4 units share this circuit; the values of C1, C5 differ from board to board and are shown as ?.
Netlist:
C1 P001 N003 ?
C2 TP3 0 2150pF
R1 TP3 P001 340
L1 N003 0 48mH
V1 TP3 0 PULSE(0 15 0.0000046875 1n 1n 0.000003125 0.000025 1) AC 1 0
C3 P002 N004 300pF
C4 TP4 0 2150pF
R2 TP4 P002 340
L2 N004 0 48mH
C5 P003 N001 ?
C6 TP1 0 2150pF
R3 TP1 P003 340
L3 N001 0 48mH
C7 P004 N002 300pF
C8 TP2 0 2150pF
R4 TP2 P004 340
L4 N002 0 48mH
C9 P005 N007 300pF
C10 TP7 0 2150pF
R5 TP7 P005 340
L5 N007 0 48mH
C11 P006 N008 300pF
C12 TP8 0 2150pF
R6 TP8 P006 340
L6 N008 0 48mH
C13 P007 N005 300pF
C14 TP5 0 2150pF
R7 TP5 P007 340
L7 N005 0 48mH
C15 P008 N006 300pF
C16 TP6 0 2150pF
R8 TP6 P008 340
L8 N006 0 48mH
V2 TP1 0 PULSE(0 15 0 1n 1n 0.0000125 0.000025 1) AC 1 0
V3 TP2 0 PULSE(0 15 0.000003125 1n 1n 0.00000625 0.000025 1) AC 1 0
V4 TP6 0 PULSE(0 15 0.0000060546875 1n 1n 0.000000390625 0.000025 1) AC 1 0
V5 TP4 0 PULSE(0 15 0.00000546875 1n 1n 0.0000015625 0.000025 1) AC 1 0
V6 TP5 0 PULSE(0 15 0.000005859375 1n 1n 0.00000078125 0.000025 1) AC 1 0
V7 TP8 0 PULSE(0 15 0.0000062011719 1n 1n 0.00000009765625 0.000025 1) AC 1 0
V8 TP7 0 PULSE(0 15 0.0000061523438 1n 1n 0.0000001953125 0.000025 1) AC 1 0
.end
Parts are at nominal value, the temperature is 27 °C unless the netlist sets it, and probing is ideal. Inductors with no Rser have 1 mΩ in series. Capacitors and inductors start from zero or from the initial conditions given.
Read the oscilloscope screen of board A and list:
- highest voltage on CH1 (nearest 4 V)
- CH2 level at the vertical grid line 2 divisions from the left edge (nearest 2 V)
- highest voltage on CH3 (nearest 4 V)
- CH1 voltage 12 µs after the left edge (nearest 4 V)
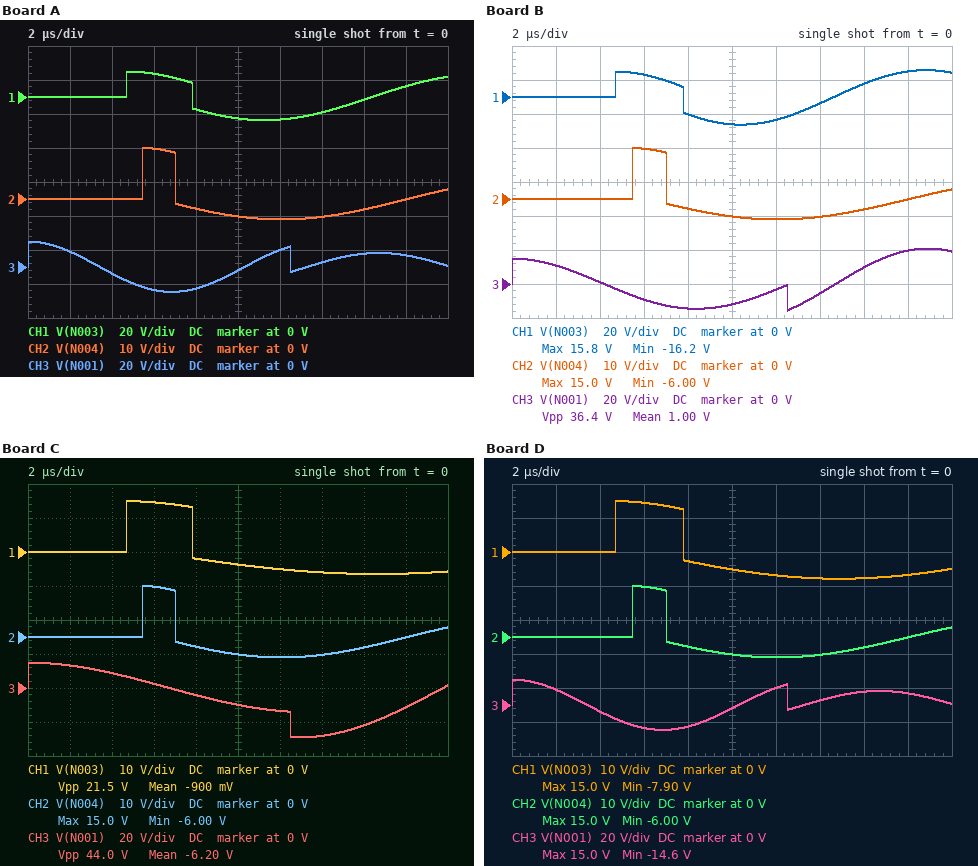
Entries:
16 V
0 V
16 V
-12 V
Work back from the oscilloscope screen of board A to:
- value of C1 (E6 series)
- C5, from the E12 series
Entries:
220 pF
100 pF
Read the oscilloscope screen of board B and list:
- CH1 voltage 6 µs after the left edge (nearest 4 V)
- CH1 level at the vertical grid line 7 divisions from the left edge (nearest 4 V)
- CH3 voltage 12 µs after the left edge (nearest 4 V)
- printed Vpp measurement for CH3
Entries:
12 V
-4 V
-4 V
36.4 V
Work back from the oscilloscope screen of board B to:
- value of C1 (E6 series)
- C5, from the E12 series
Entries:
150 pF
150 pF
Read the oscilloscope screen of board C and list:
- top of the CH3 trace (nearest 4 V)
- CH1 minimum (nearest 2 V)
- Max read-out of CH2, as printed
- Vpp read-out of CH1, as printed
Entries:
16 V
-6 V
15.0 V
21.5 V
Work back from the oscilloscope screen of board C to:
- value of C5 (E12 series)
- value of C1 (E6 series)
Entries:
390 pF
1 nF
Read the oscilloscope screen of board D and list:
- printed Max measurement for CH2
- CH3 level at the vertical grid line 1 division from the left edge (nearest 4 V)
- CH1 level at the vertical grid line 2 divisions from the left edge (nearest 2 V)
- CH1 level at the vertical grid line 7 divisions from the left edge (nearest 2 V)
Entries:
15.0 V
8 V
0 V
-8 V
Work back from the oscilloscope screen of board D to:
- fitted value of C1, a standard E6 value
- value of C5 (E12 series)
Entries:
680 pF
100 pF
